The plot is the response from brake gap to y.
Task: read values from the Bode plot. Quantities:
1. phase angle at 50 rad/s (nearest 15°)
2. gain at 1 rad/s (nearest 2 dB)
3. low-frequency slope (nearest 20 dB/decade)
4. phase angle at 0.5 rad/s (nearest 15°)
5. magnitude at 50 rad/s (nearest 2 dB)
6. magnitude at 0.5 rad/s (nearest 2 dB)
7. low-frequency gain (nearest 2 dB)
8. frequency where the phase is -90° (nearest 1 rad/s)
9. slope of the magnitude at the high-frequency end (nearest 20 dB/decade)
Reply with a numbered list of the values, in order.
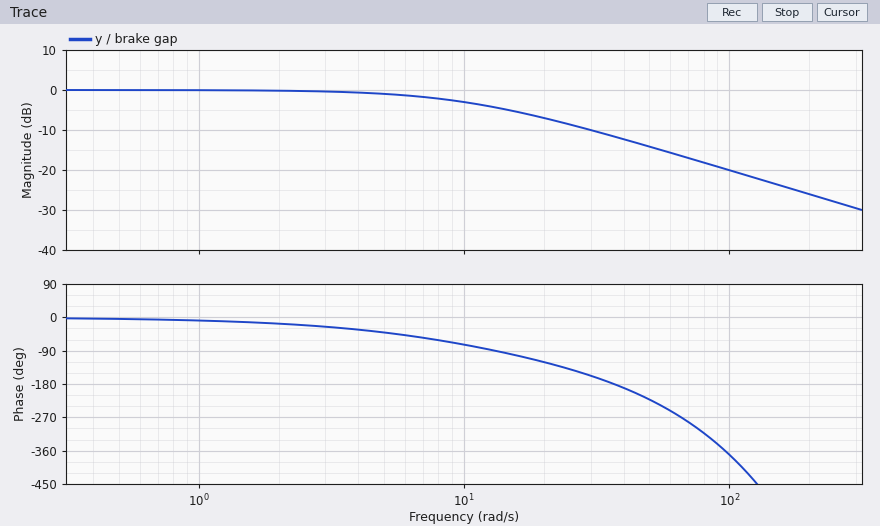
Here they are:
1. -225°
2. 0 dB
3. 0 dB/decade
4. 0°
5. -14 dB
6. 0 dB
7. 0 dB
8. 13 rad/s
9. -20 dB/decade
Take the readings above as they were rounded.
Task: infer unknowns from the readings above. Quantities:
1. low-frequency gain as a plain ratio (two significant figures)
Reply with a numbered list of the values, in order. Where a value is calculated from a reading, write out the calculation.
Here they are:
1. 10^(0 / 20) = 1.0
